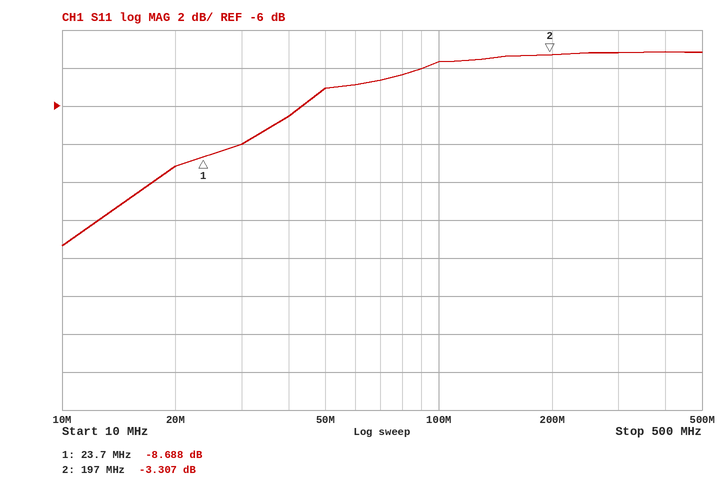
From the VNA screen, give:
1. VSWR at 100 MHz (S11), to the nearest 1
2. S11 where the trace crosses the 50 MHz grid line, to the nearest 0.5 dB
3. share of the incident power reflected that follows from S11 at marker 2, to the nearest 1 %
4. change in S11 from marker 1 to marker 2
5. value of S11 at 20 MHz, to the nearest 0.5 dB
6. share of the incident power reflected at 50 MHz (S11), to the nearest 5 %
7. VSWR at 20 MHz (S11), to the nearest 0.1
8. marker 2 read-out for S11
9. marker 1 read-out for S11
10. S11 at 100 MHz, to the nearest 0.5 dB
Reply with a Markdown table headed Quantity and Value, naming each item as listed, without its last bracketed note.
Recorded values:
| Quantity | Value |
|---|---|
| VSWR at 100 MHz (S11), to the nearest 1 | 5 |
| S11 where the trace crosses the 50 MHz grid line, to the nearest 0.5 dB | -5.0 dB |
| share of the incident power reflected that follows from S11 at marker 2, to the nearest 1 % | 47 % |
| change in S11 from marker 1 to marker 2 | 5.381 dB |
| value of S11 at 20 MHz, to the nearest 0.5 dB | -9.0 dB |
| share of the incident power reflected at 50 MHz (S11), to the nearest 5 % | 30 % |
| VSWR at 20 MHz (S11), to the nearest 0.1 | 2.1 |
| marker 2 read-out for S11 | -3.307 dB |
| marker 1 read-out for S11 | -8.688 dB |
| S11 at 100 MHz, to the nearest 0.5 dB | -3.5 dB |
